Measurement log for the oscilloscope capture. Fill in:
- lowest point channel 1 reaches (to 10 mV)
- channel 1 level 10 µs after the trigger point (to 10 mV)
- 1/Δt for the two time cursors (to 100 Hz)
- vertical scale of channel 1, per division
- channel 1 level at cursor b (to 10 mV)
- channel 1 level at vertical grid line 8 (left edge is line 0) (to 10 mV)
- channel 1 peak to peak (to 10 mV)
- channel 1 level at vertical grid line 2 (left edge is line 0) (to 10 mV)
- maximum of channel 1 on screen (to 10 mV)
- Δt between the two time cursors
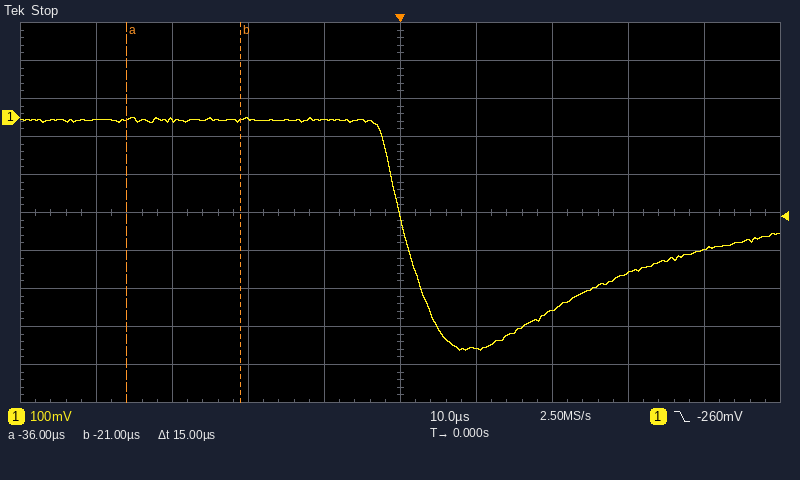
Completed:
-610 mV
-610 mV
66.7 kHz
100 mV
-10 mV
-410 mV
610 mV
-10 mV
0 mV
15 µs
